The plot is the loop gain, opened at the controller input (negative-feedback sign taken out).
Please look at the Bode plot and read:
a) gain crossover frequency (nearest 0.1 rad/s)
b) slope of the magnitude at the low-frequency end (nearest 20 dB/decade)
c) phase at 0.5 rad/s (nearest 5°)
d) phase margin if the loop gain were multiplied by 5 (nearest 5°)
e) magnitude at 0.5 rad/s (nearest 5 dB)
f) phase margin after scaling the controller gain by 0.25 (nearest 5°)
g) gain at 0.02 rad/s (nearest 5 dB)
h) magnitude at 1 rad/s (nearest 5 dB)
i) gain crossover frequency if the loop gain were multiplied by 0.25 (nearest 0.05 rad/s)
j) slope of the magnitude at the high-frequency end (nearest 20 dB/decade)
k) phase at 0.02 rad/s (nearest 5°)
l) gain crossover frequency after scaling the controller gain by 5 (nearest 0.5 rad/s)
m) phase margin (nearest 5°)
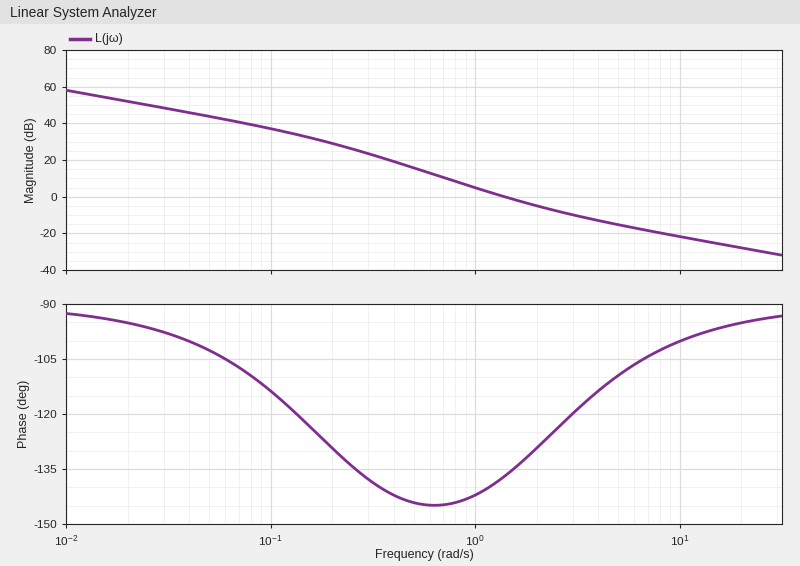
1.4 rad/s
-20 dB/decade
-145°
70°
15 dB
35°
50 dB
5 dB
0.65 rad/s
-20 dB/decade
-95°
4.5 rad/s
45°
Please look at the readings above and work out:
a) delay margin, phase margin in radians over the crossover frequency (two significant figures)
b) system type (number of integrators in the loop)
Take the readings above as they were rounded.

0.56 s
1
